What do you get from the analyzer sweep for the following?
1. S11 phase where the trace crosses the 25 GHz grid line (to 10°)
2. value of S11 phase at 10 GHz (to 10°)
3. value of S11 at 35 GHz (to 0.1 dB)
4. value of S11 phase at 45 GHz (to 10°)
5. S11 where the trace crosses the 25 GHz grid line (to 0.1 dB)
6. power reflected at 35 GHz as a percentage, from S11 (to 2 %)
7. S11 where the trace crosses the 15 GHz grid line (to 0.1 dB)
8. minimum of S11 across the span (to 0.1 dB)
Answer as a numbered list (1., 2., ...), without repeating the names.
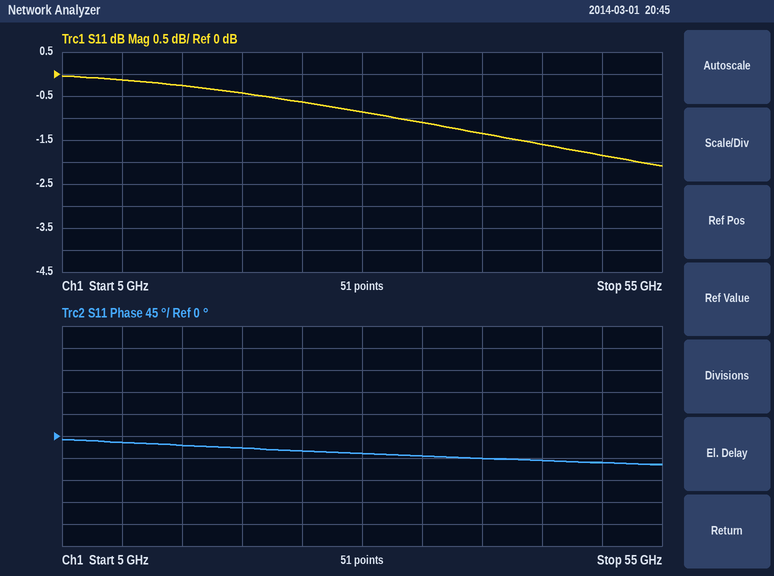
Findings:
1. -30°
2. -10°
3. -1.1 dB
4. -50°
5. -0.6 dB
6. 78 %
7. -0.3 dB
8. -2.1 dB
